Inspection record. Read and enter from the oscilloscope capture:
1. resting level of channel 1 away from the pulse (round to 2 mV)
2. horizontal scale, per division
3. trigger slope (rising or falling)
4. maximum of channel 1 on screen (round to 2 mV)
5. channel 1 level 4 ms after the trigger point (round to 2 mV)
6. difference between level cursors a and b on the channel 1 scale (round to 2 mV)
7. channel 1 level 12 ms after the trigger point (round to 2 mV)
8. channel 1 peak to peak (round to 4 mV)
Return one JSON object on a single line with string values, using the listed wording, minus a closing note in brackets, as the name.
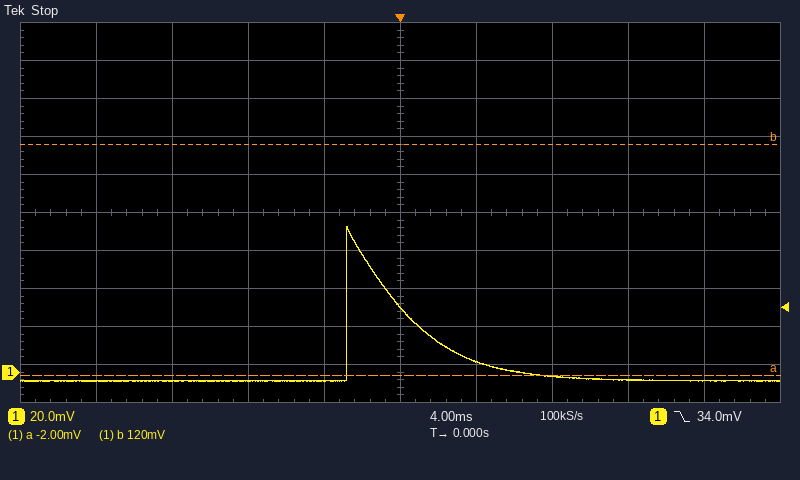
{"resting level of channel 1 away from the pulse": "-4 mV", "horizontal scale, per division": "4 ms", "trigger slope": "falling", "maximum of channel 1 on screen": "76 mV", "channel 1 level 4 ms after the trigger point": "6 mV", "difference between level cursors a and b on the channel 1 scale": "122 mV", "channel 1 level 12 ms after the trigger point": "-4 mV", "channel 1 peak to peak": "80 mV"}
